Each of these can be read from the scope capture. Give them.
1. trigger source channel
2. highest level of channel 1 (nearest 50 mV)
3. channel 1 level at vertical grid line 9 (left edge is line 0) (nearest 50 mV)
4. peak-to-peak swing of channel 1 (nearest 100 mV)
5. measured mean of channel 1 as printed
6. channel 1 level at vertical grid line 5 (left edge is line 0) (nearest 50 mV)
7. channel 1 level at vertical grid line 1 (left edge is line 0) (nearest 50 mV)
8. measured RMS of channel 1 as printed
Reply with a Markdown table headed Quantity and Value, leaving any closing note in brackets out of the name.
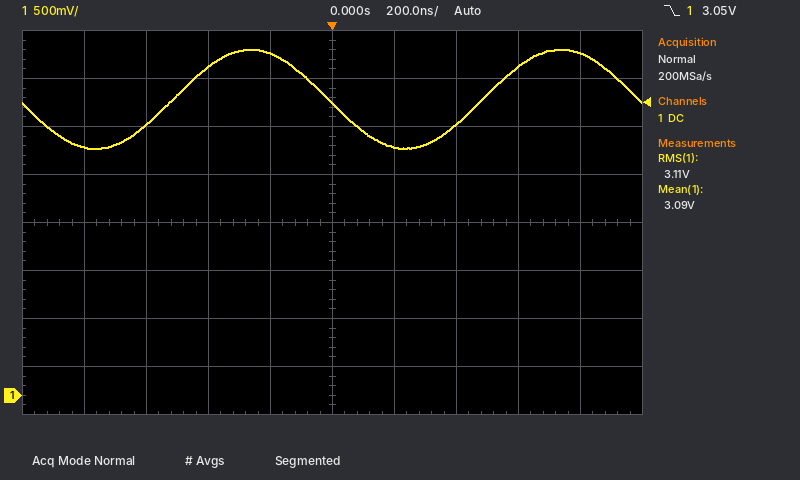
| Quantity | Value |
|---|---|
| trigger source channel | channel 1 |
| highest level of channel 1 | 3.60 V |
| channel 1 level at vertical grid line 9 (left edge is line 0) | 3.55 V |
| peak-to-peak swing of channel 1 | 1.00 V |
| measured mean of channel 1 as printed | 3.09 V |
| channel 1 level at vertical grid line 5 (left edge is line 0) | 3.05 V |
| channel 1 level at vertical grid line 1 (left edge is line 0) | 2.60 V |
| measured RMS of channel 1 as printed | 3.11 V |
